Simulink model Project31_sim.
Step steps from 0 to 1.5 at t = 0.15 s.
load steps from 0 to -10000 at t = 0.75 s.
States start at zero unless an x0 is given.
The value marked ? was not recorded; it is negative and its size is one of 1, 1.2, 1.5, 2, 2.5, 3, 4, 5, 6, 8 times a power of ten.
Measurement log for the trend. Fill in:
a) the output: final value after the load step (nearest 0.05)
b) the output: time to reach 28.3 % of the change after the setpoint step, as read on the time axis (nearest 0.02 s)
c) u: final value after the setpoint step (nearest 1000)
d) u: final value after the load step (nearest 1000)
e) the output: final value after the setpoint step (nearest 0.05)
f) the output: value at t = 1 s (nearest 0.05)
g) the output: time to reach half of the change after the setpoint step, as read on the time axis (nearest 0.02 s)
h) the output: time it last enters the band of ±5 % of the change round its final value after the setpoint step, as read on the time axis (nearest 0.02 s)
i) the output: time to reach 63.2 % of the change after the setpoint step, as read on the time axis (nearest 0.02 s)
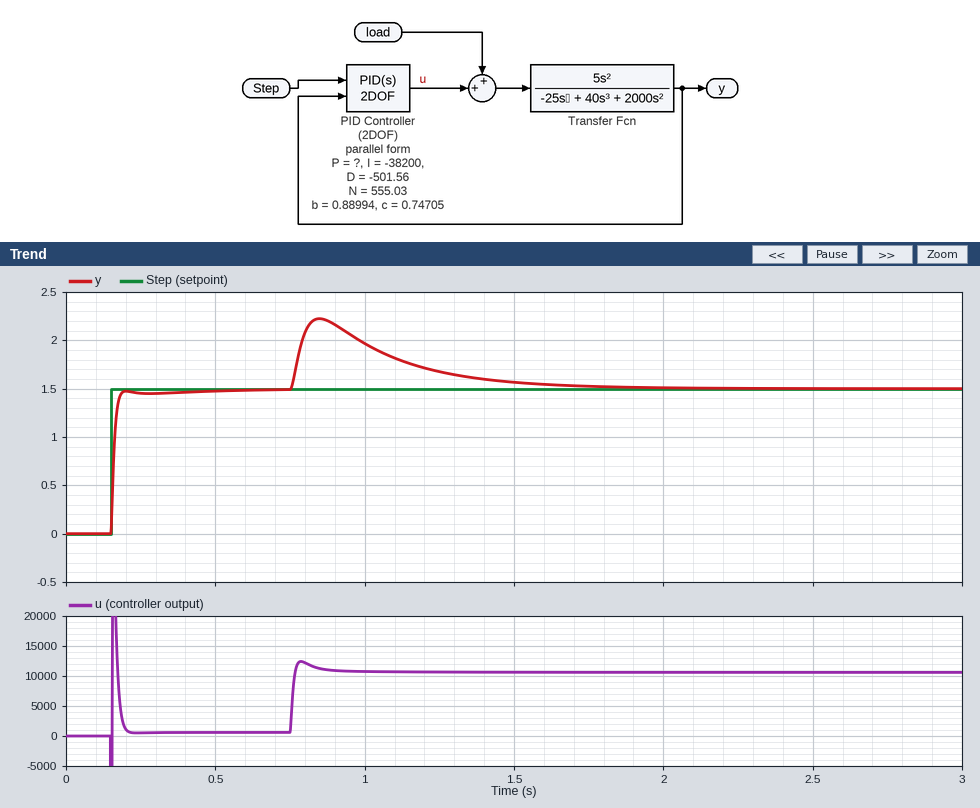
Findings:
1.50
0.16 s
1000
11000
1.50
1.95
0.16 s
0.18 s
0.16 s
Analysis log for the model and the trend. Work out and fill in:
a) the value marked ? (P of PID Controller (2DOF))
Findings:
-12000
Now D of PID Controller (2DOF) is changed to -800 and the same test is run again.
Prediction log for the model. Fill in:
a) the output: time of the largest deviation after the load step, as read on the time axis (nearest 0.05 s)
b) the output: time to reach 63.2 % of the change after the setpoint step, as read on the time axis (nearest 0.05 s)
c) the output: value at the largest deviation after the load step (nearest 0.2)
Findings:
0.90 s
0.15 s
2.2
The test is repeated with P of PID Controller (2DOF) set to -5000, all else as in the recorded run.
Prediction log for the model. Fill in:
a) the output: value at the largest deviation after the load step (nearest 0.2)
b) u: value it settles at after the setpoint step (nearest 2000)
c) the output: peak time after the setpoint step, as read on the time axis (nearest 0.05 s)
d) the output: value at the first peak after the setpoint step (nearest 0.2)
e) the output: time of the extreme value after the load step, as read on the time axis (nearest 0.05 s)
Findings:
2.8
0
0.40 s
1.6
0.90 s
